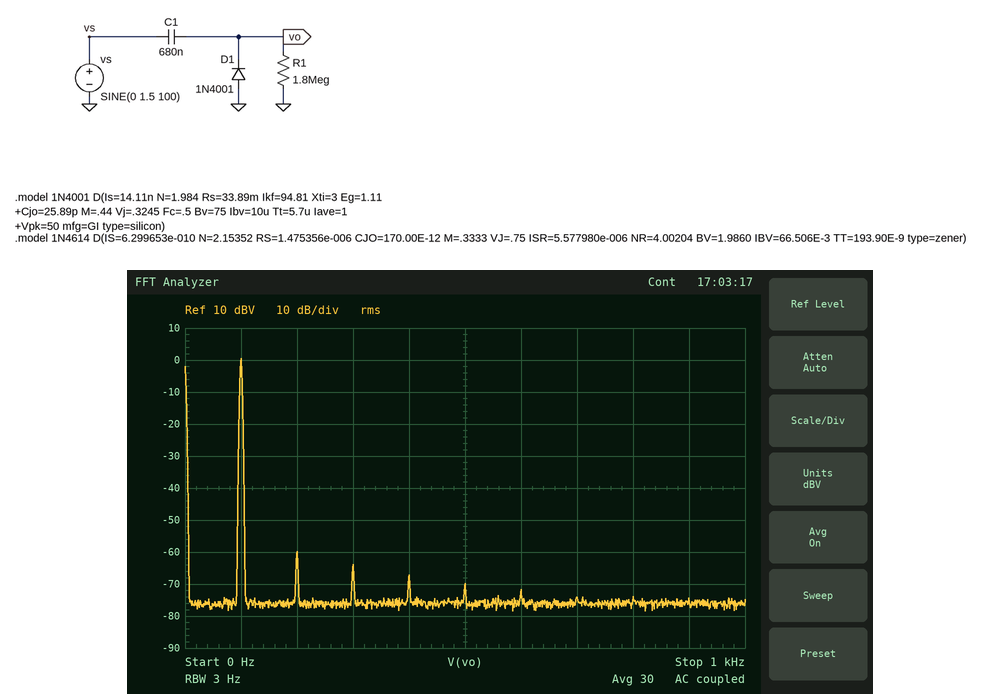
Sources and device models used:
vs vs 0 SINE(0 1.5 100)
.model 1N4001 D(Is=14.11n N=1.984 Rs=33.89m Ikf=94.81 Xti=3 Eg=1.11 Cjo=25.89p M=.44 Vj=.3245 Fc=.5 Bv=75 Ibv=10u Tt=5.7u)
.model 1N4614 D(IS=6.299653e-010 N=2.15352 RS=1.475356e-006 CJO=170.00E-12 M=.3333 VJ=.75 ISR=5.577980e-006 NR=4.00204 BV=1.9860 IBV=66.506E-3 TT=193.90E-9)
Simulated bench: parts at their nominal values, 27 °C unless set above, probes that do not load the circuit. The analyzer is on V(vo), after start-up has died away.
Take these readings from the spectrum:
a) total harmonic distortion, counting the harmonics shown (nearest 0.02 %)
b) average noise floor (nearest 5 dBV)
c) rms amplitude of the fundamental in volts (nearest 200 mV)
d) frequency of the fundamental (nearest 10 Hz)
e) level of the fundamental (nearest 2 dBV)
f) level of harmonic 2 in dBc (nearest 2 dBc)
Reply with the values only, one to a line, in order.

0.10 %
-75 dBV
1.0 V
100 Hz
0 dBV
-60 dBc
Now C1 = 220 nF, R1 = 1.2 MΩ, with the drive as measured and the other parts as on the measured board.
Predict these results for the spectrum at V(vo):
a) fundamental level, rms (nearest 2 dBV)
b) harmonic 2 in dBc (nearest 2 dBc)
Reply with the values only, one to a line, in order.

0 dBV
-48 dBc
